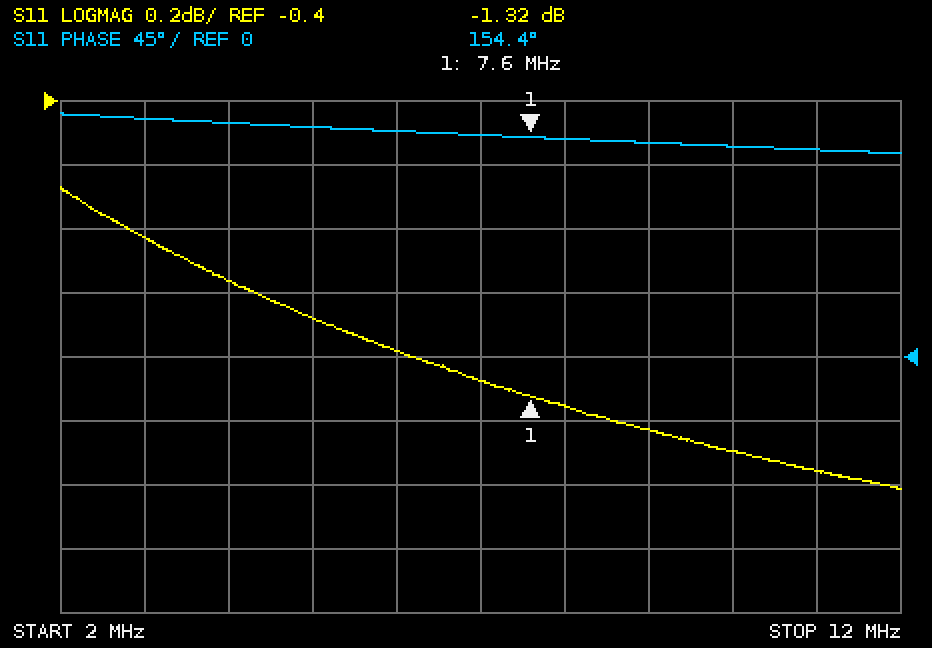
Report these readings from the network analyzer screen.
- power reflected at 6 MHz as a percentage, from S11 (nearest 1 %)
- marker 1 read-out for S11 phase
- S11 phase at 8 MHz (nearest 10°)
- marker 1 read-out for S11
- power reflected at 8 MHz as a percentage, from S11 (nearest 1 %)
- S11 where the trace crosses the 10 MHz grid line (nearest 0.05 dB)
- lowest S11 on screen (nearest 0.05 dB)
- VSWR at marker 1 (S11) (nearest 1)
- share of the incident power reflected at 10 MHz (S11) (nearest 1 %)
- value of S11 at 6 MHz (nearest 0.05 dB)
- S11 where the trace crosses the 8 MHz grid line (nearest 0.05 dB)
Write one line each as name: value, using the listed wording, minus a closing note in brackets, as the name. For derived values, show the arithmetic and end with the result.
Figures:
power reflected at 6 MHz as a percentage, from S11: 10^(-1.2/10) ≈ 76 %
marker 1 read-out for S11 phase: 154.4°
S11 phase at 8 MHz: 150°
marker 1 read-out for S11: -1.32 dB
power reflected at 8 MHz as a percentage, from S11: 10^(-1.35/10) ≈ 73 %
S11 where the trace crosses the 10 MHz grid line: -1.50 dB
lowest S11 on screen: -1.60 dB
VSWR at marker 1 (S11): (1 + 0.8590)/(1 − 0.8590) ≈ 13
share of the incident power reflected at 10 MHz (S11): 10^(-1.5/10) ≈ 71 %
value of S11 at 6 MHz: -1.20 dB
S11 where the trace crosses the 8 MHz grid line: -1.35 dB
